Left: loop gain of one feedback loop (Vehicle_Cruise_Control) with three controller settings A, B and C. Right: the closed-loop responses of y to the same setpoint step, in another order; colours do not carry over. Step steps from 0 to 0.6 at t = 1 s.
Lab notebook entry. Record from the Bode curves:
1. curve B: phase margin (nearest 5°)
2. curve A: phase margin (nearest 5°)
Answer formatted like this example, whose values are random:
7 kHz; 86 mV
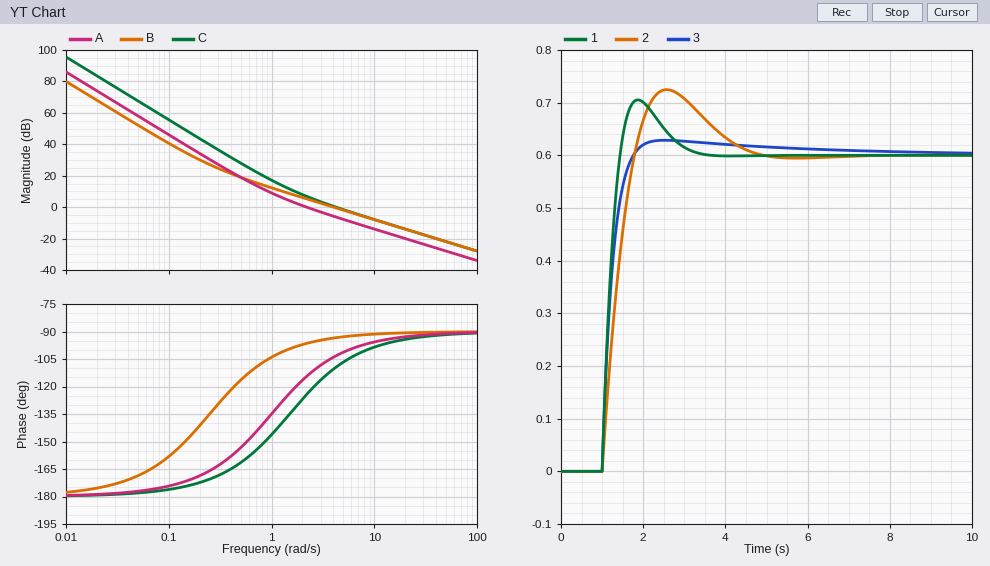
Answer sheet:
85°; 65°
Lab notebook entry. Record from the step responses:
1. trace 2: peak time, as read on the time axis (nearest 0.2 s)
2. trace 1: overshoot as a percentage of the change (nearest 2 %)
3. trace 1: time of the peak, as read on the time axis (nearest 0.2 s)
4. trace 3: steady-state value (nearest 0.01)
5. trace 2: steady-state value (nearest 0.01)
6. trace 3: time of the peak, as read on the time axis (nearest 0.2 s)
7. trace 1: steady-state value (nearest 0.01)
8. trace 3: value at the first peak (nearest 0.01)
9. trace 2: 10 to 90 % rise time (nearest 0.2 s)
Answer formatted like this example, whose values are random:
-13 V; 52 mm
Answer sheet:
2.6 s; 18 %; 1.8 s; 0.60; 0.60; 2.6 s; 0.60; 0.63; 0.6 s
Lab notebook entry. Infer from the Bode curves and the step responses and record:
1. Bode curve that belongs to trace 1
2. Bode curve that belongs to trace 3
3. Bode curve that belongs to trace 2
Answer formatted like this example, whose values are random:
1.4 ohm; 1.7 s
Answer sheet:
C; B; A
